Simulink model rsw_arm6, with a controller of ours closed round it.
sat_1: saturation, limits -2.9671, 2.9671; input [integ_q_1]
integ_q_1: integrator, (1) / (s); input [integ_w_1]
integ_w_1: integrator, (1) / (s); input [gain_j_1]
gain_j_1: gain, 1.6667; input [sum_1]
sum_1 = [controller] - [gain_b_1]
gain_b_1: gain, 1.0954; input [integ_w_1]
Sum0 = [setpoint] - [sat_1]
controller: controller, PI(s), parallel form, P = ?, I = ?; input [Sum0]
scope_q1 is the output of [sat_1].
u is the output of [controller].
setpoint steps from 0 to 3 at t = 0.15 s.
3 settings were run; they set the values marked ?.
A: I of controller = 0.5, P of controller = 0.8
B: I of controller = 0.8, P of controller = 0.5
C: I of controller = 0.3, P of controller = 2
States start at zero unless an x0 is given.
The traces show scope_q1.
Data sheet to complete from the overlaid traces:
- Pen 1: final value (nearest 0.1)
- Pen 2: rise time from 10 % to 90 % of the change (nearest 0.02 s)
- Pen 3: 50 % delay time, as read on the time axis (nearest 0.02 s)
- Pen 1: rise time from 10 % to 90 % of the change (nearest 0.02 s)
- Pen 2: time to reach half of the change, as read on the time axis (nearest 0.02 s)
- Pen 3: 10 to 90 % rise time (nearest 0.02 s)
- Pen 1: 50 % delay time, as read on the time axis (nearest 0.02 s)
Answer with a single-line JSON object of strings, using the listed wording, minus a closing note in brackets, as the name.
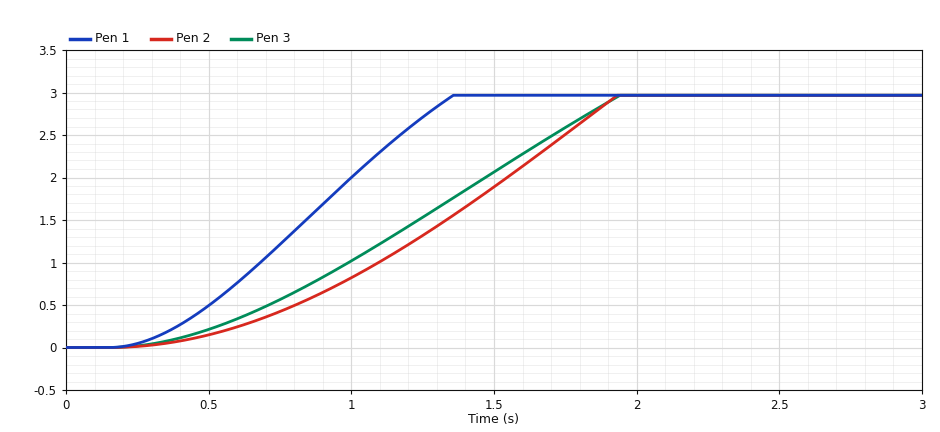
{"Pen 1: final value": "3.0", "Pen 2: rise time from 10 % to 90 % of the change": "1.16 s", "Pen 3: 50 % delay time, as read on the time axis": "1.22 s", "Pen 1: rise time from 10 % to 90 % of the change": "0.82 s", "Pen 2: time to reach half of the change, as read on the time axis": "1.32 s", "Pen 3: 10 to 90 % rise time": "1.22 s", "Pen 1: 50 % delay time, as read on the time axis": "0.84 s"}
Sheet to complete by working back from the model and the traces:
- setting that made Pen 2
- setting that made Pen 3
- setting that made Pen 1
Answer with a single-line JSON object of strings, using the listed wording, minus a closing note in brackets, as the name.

{"setting that made Pen 2": "B", "setting that made Pen 3": "A", "setting that made Pen 1": "C"}
